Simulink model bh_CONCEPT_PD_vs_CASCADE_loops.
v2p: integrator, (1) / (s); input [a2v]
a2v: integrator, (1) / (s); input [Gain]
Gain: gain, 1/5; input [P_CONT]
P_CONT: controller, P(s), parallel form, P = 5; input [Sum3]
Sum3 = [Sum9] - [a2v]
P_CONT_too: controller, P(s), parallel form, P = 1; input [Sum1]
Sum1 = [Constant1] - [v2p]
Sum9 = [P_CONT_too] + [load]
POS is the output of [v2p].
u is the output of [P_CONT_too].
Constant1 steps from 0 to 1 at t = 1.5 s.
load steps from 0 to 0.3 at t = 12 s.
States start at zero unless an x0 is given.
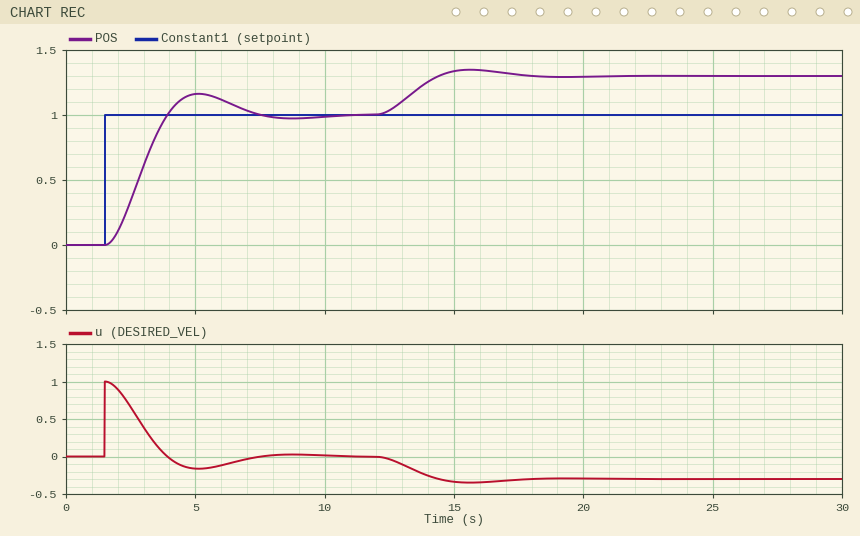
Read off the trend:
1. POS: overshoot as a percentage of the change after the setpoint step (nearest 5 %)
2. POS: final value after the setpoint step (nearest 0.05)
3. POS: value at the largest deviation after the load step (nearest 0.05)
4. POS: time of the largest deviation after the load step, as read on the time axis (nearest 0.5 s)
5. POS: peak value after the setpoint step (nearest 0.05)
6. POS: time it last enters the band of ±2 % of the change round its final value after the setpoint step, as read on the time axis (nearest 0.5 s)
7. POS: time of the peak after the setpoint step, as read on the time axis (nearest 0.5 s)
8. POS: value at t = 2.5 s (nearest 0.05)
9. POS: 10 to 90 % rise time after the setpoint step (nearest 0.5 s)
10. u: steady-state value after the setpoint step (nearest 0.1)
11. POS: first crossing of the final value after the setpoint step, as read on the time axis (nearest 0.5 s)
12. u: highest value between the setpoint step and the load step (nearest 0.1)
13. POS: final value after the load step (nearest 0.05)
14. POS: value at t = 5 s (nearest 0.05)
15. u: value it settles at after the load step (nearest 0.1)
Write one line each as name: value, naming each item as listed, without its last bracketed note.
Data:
POS: overshoot as a percentage of the change after the setpoint step: 15 %
POS: final value after the setpoint step: 1.00
POS: value at the largest deviation after the load step: 1.35
POS: time of the largest deviation after the load step, as read on the time axis: 15.5 s
POS: peak value after the setpoint step: 1.15
POS: time it last enters the band of ±2 % of the change round its final value after the setpoint step, as read on the time axis: 9.5 s
POS: time of the peak after the setpoint step, as read on the time axis: 5.0 s
POS: value at t = 2.5 s: 0.35
POS: 10 to 90 % rise time after the setpoint step: 1.5 s
u: steady-state value after the setpoint step: 0.0
POS: first crossing of the final value after the setpoint step, as read on the time axis: 4.0 s
u: highest value between the setpoint step and the load step: 1.0
POS: final value after the load step: 1.30
POS: value at t = 5 s: 1.15
u: value it settles at after the load step: -0.3
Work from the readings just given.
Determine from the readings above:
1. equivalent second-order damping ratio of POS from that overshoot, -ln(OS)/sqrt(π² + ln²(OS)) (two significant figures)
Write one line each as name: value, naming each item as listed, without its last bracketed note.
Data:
equivalent second-order damping ratio of POS from that overshoot, -ln(OS)/sqrt(π² + ln²(OS)): 0.52
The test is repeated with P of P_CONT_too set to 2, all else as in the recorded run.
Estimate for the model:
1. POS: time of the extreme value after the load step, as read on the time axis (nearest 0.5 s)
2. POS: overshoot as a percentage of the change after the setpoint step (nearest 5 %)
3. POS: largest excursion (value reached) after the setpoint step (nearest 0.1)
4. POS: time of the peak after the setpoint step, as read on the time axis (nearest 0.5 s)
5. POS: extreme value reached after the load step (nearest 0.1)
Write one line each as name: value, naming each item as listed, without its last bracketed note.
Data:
POS: time of the extreme value after the load step, as read on the time axis: 14.5 s
POS: overshoot as a percentage of the change after the setpoint step: 30 %
POS: largest excursion (value reached) after the setpoint step: 1.3
POS: time of the peak after the setpoint step, as read on the time axis: 4.0 s
POS: extreme value reached after the load step: 1.2
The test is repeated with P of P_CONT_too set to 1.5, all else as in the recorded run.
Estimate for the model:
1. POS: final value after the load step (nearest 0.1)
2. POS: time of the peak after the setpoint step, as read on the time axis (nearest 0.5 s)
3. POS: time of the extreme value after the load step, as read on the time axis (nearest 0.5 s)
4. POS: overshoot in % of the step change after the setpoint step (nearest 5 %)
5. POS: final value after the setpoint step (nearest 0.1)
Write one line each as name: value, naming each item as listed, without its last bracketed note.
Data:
POS: final value after the load step: 1.2
POS: time of the peak after the setpoint step, as read on the time axis: 4.5 s
POS: time of the extreme value after the load step, as read on the time axis: 15.0 s
POS: overshoot in % of the step change after the setpoint step: 25 %
POS: final value after the setpoint step: 1.0
